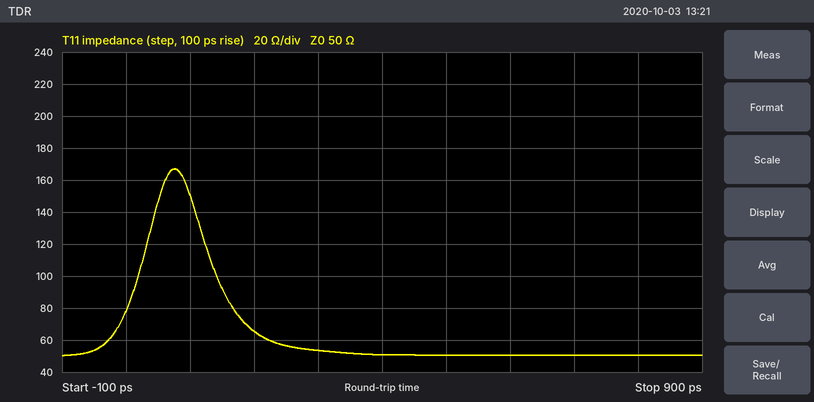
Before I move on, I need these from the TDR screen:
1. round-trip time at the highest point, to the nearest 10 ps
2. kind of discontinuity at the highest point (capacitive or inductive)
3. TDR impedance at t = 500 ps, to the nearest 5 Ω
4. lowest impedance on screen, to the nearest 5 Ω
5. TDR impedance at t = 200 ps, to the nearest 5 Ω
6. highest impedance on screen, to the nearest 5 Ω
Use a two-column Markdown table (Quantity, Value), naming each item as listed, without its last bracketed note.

| Quantity | Value |
|---|---|
| round-trip time at the highest point, to the nearest 10 ps | 80 ps |
| kind of discontinuity at the highest point | inductive |
| TDR impedance at t = 500 ps, to the nearest 5 Ω | 50 Ω |
| lowest impedance on screen, to the nearest 5 Ω | 50 Ω |
| TDR impedance at t = 200 ps, to the nearest 5 Ω | 65 Ω |
| highest impedance on screen, to the nearest 5 Ω | 165 Ω |
